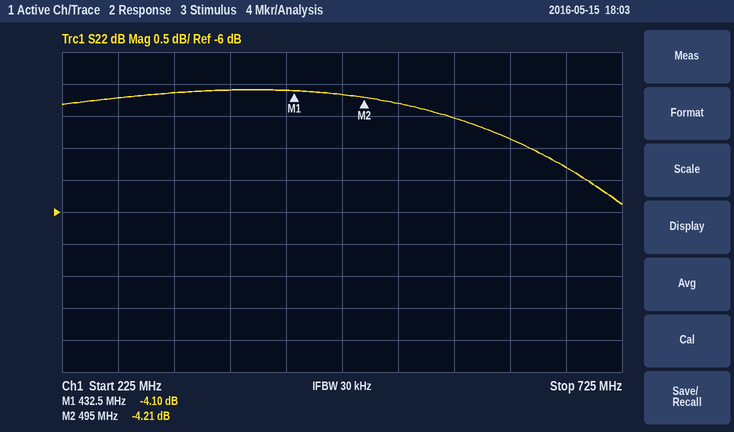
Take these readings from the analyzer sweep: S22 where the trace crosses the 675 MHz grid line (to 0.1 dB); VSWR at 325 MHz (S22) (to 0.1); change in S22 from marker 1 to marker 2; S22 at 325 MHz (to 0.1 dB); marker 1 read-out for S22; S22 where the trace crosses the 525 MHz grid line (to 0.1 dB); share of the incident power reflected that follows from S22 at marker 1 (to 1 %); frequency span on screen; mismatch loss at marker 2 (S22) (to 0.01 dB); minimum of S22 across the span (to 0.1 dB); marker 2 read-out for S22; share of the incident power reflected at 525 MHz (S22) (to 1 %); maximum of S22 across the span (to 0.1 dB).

-5.3 dB
4.3
-0.11 dB
-4.1 dB
-4.10 dB
-4.3 dB
39 %
500 MHz
2.07 dB
-5.9 dB
-4.21 dB
37 %
-4.1 dB
